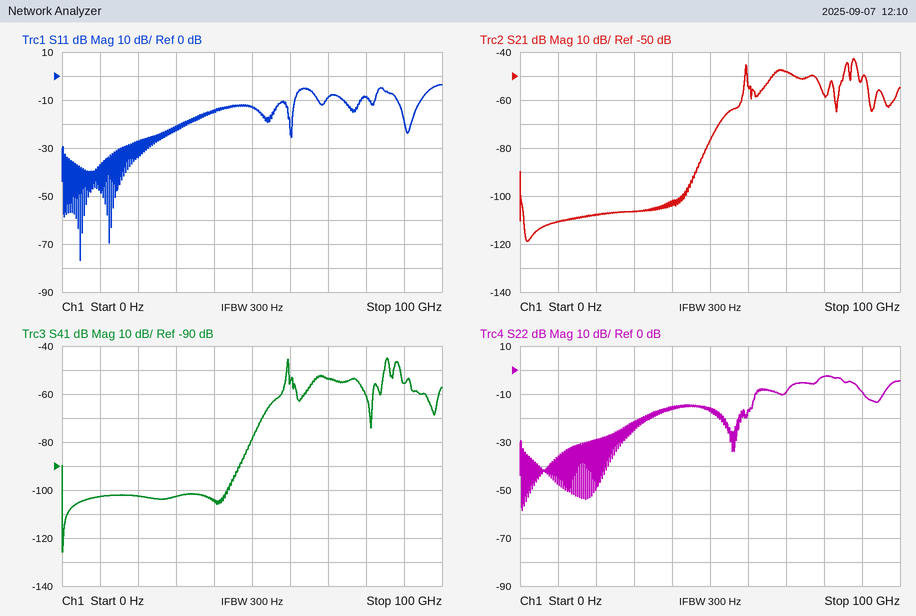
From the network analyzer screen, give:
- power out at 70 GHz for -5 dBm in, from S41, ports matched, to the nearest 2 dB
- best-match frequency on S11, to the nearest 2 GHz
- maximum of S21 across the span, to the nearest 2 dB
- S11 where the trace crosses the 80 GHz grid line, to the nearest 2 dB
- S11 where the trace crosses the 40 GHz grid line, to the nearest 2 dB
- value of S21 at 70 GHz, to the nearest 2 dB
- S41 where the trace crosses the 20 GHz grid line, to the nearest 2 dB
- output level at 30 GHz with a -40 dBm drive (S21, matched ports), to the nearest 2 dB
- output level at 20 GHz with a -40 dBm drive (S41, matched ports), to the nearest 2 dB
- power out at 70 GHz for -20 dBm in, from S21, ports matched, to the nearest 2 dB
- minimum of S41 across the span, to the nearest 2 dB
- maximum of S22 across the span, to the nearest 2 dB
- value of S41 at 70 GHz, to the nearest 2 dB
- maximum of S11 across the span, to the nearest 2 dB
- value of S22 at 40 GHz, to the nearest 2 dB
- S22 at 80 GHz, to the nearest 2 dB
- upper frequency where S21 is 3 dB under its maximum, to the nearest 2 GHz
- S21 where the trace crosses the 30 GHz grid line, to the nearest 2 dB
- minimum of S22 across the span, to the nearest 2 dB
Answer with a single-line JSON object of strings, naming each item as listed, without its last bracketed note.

{"power out at 70 GHz for -5 dBm in, from S41, ports matched, to the nearest 2 dB": "-58 dBm", "best-match frequency on S11, to the nearest 2 GHz": "4 GHz", "maximum of S21 across the span, to the nearest 2 dB": "-42 dB", "S11 where the trace crosses the 80 GHz grid line, to the nearest 2 dB": "-8 dB", "S11 where the trace crosses the 40 GHz grid line, to the nearest 2 dB": "-14 dB", "value of S21 at 70 GHz, to the nearest 2 dB": "-48 dB", "S41 where the trace crosses the 20 GHz grid line, to the nearest 2 dB": "-102 dB", "output level at 30 GHz with a -40 dBm drive (S21, matched ports), to the nearest 2 dB": "-146 dBm", "output level at 20 GHz with a -40 dBm drive (S41, matched ports), to the nearest 2 dB": "-142 dBm", "power out at 70 GHz for -20 dBm in, from S21, ports matched, to the nearest 2 dB": "-68 dBm", "minimum of S41 across the span, to the nearest 2 dB": "-126 dB", "maximum of S22 across the span, to the nearest 2 dB": "-2 dB", "value of S41 at 70 GHz, to the nearest 2 dB": "-54 dB", "maximum of S11 across the span, to the nearest 2 dB": "-4 dB", "value of S22 at 40 GHz, to the nearest 2 dB": "-16 dB", "S22 at 80 GHz, to the nearest 2 dB": "-2 dB", "upper frequency where S21 is 3 dB under its maximum, to the nearest 2 GHz": "88 GHz", "S21 where the trace crosses the 30 GHz grid line, to the nearest 2 dB": "-106 dB", "minimum of S22 across the span, to the nearest 2 dB": "-58 dB"}
